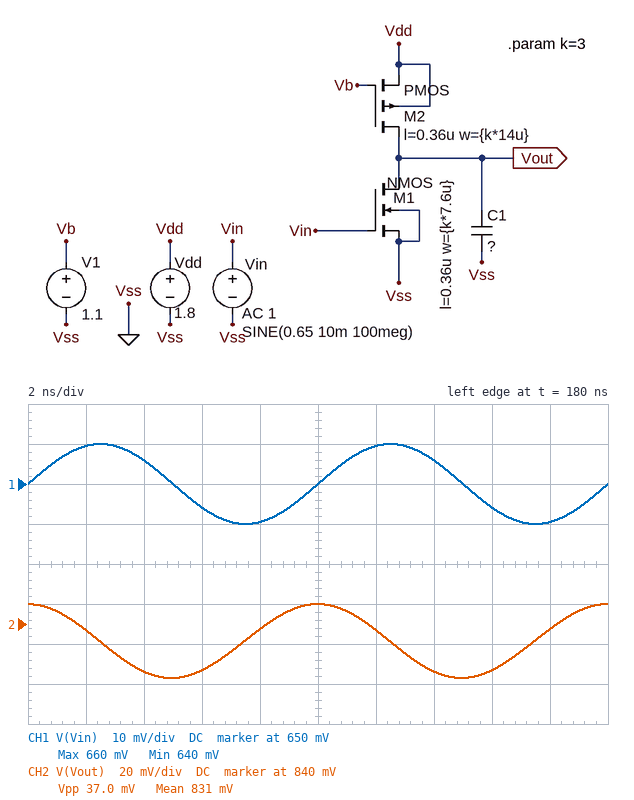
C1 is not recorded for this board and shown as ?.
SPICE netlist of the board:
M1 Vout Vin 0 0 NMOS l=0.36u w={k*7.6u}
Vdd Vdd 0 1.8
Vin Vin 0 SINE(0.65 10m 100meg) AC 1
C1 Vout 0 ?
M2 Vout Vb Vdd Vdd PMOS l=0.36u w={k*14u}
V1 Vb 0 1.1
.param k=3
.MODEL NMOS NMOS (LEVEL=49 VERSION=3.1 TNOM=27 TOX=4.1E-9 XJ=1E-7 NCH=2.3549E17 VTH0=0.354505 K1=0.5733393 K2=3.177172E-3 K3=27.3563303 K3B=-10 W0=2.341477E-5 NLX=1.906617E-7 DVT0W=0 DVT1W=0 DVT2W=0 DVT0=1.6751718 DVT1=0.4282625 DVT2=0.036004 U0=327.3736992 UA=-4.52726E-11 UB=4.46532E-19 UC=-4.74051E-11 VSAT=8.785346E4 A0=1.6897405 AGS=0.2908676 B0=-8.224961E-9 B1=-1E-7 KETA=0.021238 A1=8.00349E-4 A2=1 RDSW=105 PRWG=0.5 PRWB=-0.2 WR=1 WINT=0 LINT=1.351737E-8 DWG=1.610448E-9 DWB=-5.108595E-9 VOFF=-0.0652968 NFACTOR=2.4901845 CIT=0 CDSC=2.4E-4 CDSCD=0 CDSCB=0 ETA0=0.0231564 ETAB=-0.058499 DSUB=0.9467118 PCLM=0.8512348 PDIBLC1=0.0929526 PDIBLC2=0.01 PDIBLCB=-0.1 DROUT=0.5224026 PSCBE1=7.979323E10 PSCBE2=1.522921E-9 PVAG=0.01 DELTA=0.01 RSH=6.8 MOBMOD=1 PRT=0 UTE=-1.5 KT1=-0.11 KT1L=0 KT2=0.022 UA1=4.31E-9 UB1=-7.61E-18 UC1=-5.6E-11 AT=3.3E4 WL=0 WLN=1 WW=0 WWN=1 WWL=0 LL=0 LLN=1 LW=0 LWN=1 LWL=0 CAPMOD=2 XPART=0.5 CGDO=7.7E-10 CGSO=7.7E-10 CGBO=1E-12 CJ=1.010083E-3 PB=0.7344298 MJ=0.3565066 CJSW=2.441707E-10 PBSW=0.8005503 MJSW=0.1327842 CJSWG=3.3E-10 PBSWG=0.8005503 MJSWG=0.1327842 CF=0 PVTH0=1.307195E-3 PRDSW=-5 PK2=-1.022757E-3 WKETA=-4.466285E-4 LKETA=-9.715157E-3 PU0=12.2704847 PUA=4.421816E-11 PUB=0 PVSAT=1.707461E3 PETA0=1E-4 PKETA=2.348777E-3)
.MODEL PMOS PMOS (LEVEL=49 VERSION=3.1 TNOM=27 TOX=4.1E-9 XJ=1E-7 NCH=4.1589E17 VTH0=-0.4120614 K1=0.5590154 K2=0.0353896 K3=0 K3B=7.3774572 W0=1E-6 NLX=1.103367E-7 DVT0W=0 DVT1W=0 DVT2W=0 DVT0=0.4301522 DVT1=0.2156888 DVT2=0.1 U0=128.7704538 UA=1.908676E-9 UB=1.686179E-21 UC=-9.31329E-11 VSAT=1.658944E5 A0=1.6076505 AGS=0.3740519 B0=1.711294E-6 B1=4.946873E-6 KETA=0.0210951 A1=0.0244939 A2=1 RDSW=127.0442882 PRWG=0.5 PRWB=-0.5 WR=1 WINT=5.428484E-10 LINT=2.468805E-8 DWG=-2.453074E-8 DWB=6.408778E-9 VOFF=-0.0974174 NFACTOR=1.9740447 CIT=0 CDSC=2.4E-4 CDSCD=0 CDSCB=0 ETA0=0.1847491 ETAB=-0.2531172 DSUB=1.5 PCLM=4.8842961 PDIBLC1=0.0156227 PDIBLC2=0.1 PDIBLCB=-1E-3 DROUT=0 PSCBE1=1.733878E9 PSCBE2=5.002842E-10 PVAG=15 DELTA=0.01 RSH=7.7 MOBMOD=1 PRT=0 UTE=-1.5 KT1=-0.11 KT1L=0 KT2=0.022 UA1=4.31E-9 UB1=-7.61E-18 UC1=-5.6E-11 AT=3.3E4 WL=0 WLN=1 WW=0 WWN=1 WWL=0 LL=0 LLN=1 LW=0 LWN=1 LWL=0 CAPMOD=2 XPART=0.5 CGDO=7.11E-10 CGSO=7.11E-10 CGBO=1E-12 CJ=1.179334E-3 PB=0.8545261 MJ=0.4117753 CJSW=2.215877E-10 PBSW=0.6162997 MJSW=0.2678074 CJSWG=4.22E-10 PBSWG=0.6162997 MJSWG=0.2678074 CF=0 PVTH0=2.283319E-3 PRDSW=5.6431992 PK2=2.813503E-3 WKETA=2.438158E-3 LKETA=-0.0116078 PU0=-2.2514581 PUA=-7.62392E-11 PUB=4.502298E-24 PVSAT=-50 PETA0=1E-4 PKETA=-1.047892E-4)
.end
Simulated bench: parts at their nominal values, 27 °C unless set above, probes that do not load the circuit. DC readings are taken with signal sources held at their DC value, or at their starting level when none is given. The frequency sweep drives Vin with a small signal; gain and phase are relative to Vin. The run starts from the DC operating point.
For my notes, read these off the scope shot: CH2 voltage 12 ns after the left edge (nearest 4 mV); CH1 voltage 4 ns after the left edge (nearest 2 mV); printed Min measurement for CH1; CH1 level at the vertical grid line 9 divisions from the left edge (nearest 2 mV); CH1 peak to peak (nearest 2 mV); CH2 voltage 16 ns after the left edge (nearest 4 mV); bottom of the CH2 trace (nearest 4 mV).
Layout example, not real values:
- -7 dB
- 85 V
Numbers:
- 836 mV
- 656 mV
- 640 mV
- 640 mV
- 20 mV
- 816 mV
- 812 mV
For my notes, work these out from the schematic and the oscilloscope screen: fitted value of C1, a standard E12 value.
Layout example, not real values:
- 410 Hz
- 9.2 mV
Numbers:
- 2.2 pF
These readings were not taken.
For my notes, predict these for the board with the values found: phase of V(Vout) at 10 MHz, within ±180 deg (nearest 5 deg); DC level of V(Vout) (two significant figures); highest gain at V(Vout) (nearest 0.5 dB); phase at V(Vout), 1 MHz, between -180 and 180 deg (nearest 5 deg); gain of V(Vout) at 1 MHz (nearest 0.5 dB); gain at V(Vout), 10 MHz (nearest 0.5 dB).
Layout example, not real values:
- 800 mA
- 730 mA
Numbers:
- 105 deg
- 840 mV
- 36.0 dB
- 160 deg
- 35.5 dB
- 25.0 dB
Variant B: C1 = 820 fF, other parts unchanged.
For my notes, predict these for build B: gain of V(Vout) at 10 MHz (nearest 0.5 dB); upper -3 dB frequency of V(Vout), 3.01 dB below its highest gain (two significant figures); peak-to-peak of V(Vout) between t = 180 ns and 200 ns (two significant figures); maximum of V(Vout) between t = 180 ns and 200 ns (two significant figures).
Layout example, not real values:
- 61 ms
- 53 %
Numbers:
- 31.5 dB
- 7.7 MHz
- 94 mV
- 880 mV
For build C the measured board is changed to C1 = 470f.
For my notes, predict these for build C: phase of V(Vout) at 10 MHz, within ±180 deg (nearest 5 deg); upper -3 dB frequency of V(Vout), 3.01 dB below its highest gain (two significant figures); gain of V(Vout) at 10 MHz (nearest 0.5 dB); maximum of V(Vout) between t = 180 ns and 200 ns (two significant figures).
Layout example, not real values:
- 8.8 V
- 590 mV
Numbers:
- 140 deg
- 13 MHz
- 33.5 dB
- 910 mV
